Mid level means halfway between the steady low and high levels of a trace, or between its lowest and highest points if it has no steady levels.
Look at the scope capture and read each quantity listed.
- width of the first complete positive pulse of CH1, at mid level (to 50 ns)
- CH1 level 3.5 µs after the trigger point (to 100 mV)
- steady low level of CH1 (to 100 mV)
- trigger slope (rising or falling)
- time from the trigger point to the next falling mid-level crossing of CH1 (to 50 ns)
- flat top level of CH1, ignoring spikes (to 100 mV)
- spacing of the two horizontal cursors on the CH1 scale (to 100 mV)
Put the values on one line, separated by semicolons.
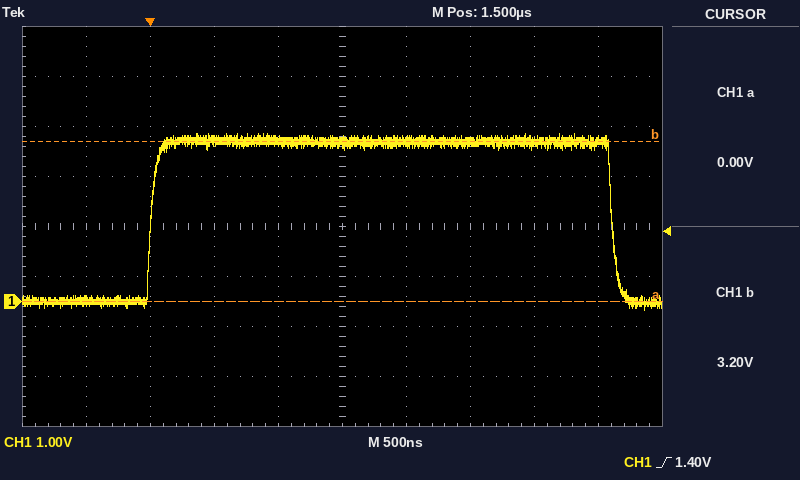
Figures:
3.60 µs; 3.2 V; 0.0 V; rising; 3.60 µs; 3.2 V; 3.2 V
